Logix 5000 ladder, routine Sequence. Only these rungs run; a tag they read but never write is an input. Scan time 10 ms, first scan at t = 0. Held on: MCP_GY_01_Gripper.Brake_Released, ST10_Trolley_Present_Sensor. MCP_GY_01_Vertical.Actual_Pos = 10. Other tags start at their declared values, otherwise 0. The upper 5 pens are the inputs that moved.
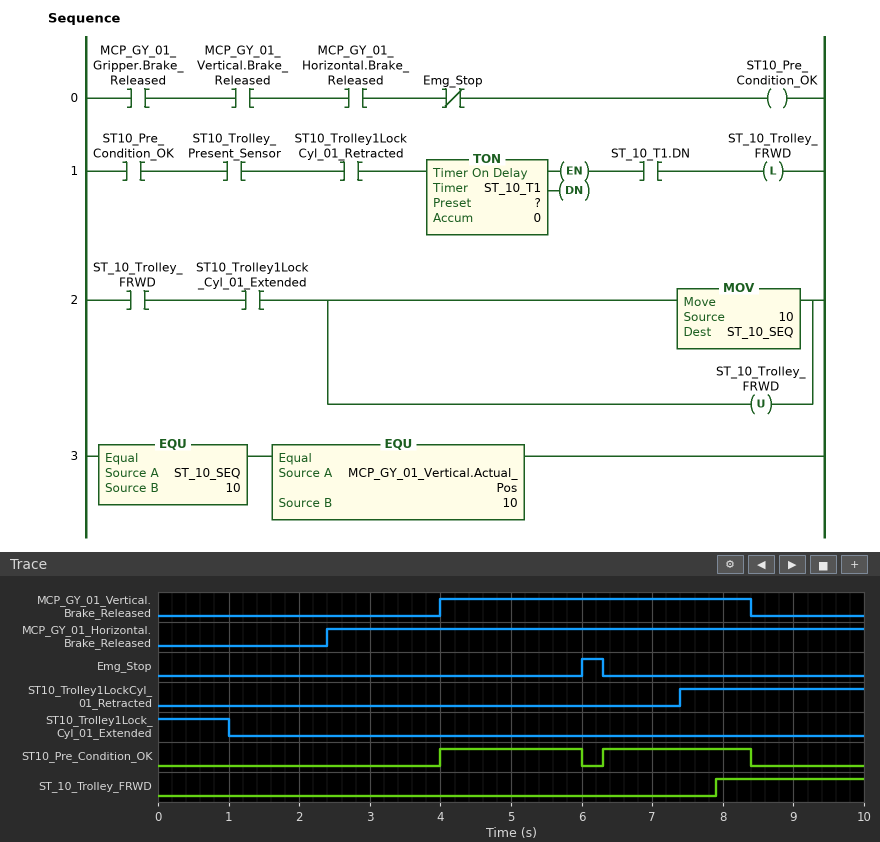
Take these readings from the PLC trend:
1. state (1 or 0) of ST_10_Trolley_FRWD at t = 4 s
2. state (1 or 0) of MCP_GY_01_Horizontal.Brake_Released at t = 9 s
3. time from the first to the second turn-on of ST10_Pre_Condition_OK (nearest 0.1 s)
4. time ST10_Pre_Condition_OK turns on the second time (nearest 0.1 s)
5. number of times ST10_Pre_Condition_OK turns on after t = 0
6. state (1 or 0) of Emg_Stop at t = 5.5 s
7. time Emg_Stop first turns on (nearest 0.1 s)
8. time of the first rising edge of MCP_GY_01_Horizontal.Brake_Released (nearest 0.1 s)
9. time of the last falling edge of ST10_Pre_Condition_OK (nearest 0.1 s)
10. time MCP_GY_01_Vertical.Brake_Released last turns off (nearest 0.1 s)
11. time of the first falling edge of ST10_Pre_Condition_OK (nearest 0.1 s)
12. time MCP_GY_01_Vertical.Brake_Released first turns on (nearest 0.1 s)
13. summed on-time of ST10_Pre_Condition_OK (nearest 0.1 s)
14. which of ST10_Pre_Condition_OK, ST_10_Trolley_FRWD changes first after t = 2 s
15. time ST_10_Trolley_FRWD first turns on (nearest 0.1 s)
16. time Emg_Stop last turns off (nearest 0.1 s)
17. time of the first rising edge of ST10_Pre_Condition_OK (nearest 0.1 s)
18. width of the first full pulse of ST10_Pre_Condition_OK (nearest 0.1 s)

0
1
2.3 s
6.3 s
2
0
6.0 s
2.4 s
8.4 s
8.4 s
6.0 s
4.0 s
4.1 s
ST10_Pre_Condition_OK
7.9 s
6.3 s
4.0 s
2.0 s
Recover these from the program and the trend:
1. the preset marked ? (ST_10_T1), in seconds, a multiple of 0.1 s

0.5 s
